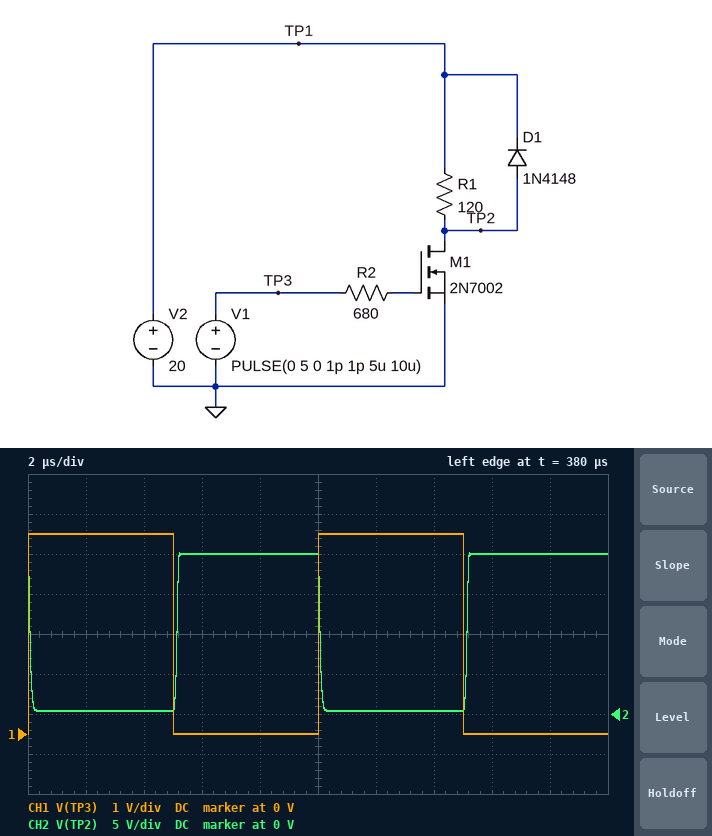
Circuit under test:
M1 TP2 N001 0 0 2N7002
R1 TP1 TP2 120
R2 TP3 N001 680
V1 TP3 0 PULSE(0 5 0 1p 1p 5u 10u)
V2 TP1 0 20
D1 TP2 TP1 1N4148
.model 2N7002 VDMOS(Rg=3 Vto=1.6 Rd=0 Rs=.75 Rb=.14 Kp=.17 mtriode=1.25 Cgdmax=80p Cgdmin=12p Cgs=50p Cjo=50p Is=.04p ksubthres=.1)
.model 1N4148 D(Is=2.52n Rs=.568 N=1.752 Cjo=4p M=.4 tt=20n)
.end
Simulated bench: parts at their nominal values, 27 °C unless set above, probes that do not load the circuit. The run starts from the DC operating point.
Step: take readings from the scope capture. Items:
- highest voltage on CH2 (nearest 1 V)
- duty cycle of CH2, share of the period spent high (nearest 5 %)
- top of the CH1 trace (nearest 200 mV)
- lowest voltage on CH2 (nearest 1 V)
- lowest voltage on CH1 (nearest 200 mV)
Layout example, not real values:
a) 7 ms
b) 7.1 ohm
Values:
a) 20 V
b) 50 %
c) 5.0 V
d) 0 V
e) 0 V
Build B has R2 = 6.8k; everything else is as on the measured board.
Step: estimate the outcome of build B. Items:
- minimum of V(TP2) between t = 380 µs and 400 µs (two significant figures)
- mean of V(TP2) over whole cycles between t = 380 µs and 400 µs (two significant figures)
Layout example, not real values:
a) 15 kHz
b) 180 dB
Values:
a) 370 mV
b) 9.2 V
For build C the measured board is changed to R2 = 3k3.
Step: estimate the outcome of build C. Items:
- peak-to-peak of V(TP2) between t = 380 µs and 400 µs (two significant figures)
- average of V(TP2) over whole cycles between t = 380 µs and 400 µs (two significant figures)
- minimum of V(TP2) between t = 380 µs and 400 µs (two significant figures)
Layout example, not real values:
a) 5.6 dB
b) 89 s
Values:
a) 20 V
b) 9.7 V
c) 370 mV
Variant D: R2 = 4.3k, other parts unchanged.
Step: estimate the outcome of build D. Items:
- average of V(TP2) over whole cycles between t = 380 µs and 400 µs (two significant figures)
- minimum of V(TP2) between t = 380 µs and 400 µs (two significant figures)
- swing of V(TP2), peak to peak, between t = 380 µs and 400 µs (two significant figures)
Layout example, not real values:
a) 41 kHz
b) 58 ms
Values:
a) 9.6 V
b) 370 mV
c) 20 V
